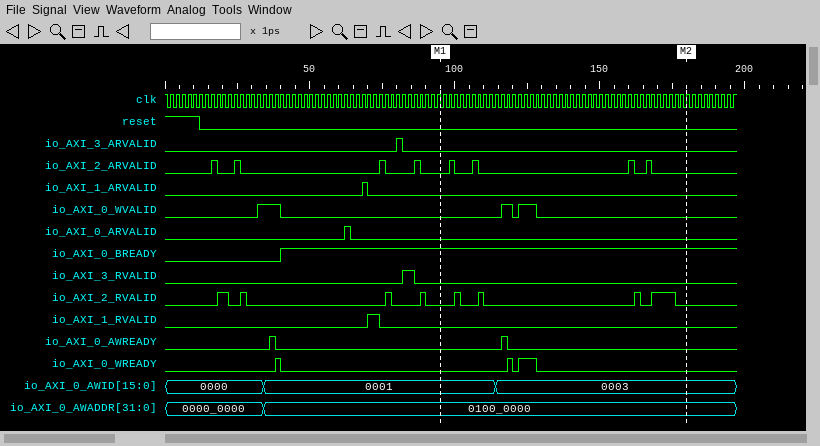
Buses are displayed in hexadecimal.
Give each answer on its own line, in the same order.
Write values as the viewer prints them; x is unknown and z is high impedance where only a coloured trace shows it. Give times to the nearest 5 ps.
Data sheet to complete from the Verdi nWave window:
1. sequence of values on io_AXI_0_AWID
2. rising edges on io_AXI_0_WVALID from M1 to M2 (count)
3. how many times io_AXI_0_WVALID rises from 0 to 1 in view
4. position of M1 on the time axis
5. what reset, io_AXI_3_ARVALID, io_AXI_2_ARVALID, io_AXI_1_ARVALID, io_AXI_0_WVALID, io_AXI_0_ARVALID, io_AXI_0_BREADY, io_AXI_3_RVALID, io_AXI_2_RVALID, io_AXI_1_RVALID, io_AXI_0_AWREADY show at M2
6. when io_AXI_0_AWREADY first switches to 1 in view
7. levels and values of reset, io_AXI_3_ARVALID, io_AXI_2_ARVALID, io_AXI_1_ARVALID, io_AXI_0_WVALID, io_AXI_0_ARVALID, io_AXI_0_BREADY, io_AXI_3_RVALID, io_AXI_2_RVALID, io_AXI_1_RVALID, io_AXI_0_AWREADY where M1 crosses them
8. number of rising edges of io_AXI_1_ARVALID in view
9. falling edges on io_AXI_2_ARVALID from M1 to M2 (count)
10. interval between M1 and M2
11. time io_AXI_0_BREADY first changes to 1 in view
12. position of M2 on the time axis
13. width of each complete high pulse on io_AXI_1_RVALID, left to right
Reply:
0000, 0001, 0003
2
3
95 ps
reset=0, io_AXI_3_ARVALID=0, io_AXI_2_ARVALID=0, io_AXI_1_ARVALID=0, io_AXI_0_WVALID=0, io_AXI_0_ARVALID=0, io_AXI_0_BREADY=1, io_AXI_3_RVALID=0, io_AXI_2_RVALID=0, io_AXI_1_RVALID=0, io_AXI_0_AWREADY=0
35 ps
reset=0, io_AXI_3_ARVALID=0, io_AXI_2_ARVALID=0, io_AXI_1_ARVALID=0, io_AXI_0_WVALID=0, io_AXI_0_ARVALID=0, io_AXI_0_BREADY=1, io_AXI_3_RVALID=0, io_AXI_2_RVALID=0, io_AXI_1_RVALID=0, io_AXI_0_AWREADY=0
1
4
85 ps
40 ps
180 ps
5 ps
